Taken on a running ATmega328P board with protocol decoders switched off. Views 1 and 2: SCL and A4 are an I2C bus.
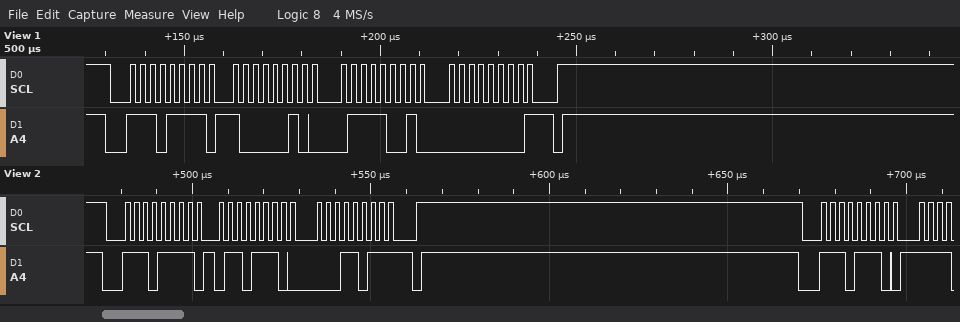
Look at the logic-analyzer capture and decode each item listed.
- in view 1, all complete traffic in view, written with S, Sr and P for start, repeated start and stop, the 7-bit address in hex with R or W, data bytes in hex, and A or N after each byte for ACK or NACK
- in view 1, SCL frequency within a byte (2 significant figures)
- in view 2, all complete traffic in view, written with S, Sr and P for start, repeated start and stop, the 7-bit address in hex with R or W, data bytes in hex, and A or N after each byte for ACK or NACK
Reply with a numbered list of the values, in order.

1. S 77R A 82 A 79 A 00 N P
2. 400 kHz
3. S 77R A 6E A 1B N P S 77W A
